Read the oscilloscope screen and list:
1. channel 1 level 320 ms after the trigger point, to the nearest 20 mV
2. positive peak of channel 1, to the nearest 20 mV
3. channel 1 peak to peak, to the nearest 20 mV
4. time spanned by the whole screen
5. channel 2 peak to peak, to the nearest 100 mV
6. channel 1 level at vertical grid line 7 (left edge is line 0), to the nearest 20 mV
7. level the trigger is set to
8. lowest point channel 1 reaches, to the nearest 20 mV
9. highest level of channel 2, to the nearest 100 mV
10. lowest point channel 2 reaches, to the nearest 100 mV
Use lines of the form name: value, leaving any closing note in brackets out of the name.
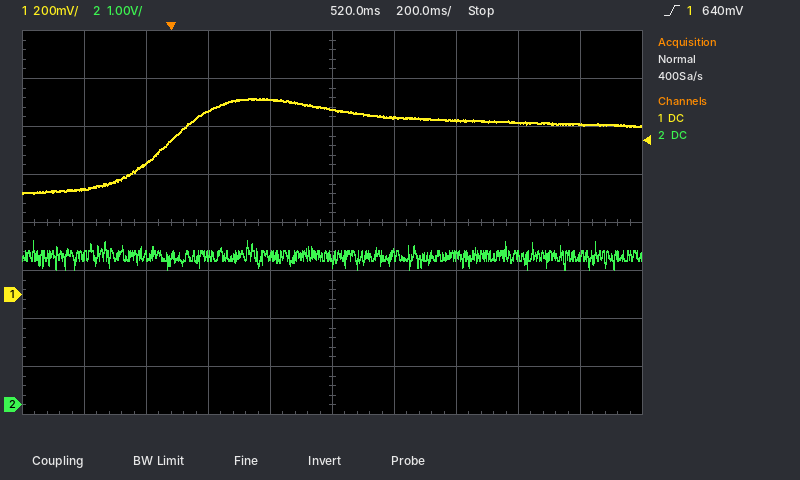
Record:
channel 1 level 320 ms after the trigger point, to the nearest 20 mV: 820 mV
positive peak of channel 1, to the nearest 20 mV: 820 mV
channel 1 peak to peak, to the nearest 20 mV: 400 mV
time spanned by the whole screen: 2 s
channel 2 peak to peak, to the nearest 100 mV: 600 mV
channel 1 level at vertical grid line 7 (left edge is line 0), to the nearest 20 mV: 720 mV
level the trigger is set to: 640 mV
lowest point channel 1 reaches, to the nearest 20 mV: 420 mV
highest level of channel 2, to the nearest 100 mV: 3.4 V
lowest point channel 2 reaches, to the nearest 100 mV: 2.8 V
